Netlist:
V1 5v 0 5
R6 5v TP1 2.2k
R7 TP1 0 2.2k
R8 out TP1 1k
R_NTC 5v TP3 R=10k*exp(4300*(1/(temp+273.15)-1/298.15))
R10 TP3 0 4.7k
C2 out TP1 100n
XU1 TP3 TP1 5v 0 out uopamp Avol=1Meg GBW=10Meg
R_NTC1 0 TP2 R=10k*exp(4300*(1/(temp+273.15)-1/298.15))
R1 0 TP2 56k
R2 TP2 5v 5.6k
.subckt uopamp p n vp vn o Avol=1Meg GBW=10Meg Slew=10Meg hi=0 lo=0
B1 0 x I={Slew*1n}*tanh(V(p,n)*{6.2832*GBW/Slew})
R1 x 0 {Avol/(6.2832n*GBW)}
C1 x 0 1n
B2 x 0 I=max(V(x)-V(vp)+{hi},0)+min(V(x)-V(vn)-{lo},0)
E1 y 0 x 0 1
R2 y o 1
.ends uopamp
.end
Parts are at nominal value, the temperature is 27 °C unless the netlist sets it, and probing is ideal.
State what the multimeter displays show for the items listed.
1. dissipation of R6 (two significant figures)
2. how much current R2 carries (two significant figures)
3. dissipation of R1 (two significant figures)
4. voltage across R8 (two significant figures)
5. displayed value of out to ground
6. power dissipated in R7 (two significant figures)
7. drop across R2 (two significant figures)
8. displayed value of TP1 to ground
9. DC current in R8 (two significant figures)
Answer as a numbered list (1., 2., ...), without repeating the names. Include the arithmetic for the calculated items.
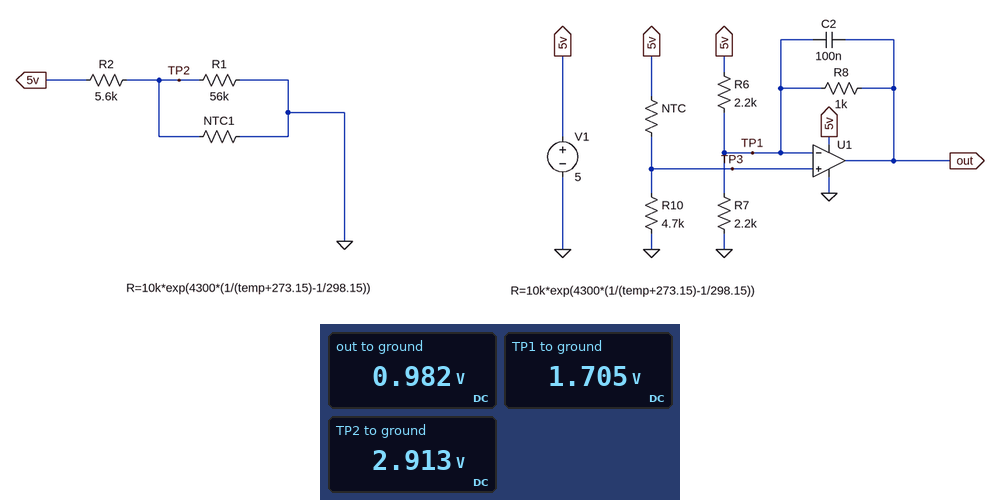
1. (5 V - 1.705 V)^2 / 2.2 kΩ = 4.9 mW
2. (5 V - 2.913 V) / 5.6 kΩ = 370 µA
3. (2.913 V)^2 / 56 kΩ = 150 µW
4. 1.705 V - 982 mV = 720 mV
5. 0.982 V
6. (1.705 V)^2 / 2.2 kΩ = 1.3 mW
7. 5 V - 2.913 V = 2.1 V
8. 1.705 V
9. (1.705 V - 982 mV) / 1 kΩ = 720 µA
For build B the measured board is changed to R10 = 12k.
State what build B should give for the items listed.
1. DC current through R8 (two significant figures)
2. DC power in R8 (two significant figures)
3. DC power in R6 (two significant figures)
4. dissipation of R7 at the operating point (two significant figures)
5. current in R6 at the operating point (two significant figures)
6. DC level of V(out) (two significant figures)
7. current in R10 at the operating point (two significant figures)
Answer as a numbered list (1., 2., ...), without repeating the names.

1. 310 µA
2. 99 µW
3. 2.1 mW
4. 3.7 mW
5. 980 µA
6. 3.2 V
7. 240 µA
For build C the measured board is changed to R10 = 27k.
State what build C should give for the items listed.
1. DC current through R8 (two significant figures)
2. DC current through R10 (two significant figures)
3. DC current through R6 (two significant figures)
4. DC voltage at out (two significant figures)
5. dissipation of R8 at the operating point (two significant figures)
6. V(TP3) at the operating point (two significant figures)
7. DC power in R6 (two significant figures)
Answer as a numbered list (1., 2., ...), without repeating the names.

1. 1.1 mA
2. 140 µA
3. 570 µA
4. 4.9 V
5. 1.3 mW
6. 3.7 V
7. 720 µW
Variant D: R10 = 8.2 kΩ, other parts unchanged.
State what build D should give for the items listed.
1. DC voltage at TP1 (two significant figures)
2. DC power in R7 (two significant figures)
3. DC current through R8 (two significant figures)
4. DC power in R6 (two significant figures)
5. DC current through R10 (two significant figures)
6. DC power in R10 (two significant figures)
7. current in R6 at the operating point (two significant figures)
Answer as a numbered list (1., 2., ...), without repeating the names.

1. 2.4 V
2. 2.6 mW
3. 120 µA
4. 3.1 mW
5. 290 µA
6. 690 µW
7. 1.2 mA
